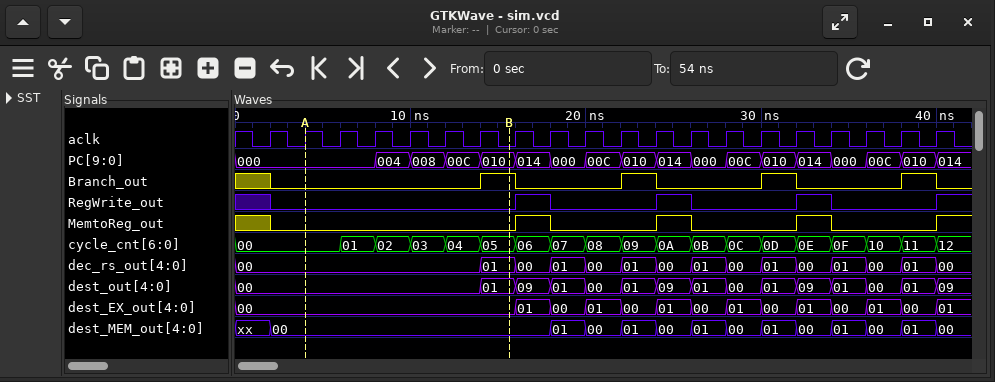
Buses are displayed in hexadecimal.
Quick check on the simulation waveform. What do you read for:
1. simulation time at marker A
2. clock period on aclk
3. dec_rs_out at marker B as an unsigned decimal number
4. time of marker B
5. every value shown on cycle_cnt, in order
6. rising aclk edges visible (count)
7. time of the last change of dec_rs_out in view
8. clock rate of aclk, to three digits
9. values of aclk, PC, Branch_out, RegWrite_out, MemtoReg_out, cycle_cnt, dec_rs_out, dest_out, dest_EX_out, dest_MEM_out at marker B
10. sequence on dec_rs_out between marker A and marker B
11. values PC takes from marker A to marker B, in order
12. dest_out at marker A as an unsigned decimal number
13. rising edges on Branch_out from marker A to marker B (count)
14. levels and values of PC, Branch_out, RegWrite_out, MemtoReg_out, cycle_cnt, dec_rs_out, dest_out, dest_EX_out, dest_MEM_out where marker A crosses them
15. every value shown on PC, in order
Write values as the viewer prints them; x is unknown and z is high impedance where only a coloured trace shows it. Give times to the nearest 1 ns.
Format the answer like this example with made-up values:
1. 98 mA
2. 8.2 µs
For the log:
1. 4 ns
2. 2 ns
3. 1
4. 16 ns
5. 00, 01, 02, 03, 04, 05, 06, 07, 08, 09, 0A, 0B, 0C, 0D, 0E, 0F, 10, 11, 12
6. 20
7. 40 ns
8. 500 MHz
9. aclk=0, PC=010, Branch_out=1, RegWrite_out=0, MemtoReg_out=0, cycle_cnt=05, dec_rs_out=01, dest_out=01, dest_EX_out=00, dest_MEM_out=00
10. 00, 01
11. 000, 004, 008, 00C, 010
12. 0
13. 1
14. PC=000, Branch_out=0, RegWrite_out=0, MemtoReg_out=0, cycle_cnt=00, dec_rs_out=00, dest_out=00, dest_EX_out=00, dest_MEM_out=00
15. 000, 004, 008, 00C, 010, 014, 000, 00C, 010, 014, 000, 00C, 010, 014, 000, 00C, 010, 014
